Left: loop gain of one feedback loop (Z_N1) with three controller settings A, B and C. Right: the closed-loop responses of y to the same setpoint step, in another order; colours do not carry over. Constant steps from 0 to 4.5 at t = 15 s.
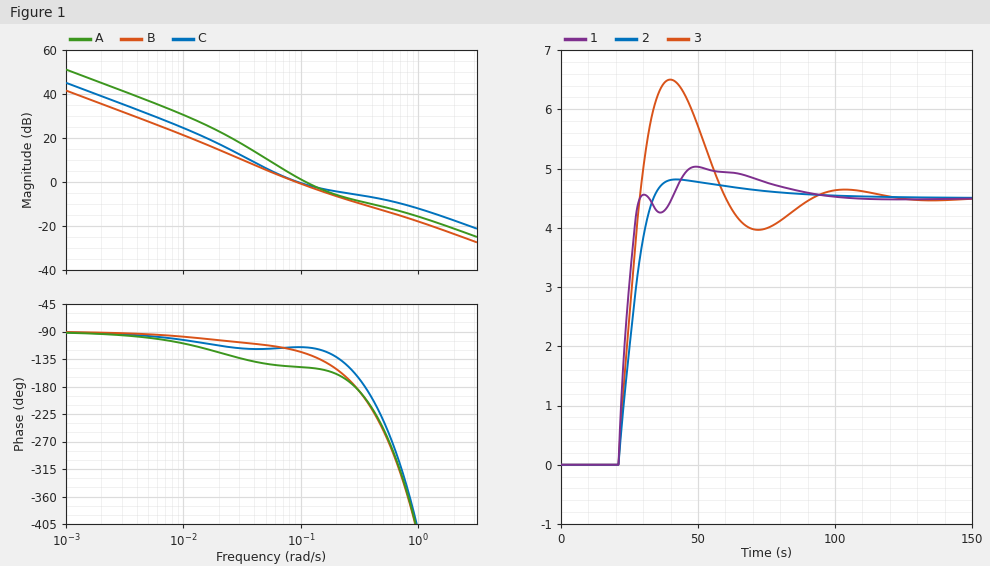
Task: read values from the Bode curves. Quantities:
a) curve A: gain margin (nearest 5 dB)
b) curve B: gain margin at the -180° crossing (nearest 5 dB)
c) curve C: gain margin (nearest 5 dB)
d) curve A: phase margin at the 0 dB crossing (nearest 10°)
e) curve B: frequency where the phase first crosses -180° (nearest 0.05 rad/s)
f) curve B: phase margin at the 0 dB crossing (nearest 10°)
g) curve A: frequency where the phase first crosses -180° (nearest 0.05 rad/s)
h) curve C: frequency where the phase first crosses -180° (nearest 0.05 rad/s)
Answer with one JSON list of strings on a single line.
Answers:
["10 dB", "10 dB", "5 dB", "30°", "0.30 rad/s", "60°", "0.30 rad/s", "0.35 rad/s"]
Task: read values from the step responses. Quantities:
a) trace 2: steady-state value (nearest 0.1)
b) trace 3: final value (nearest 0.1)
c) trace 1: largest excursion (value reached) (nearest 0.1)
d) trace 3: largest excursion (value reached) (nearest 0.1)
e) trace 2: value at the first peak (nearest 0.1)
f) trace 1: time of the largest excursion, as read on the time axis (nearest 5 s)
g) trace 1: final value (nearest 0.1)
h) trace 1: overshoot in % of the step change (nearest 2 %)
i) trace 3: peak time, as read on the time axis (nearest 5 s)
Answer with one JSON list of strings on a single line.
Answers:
["4.5", "4.5", "5.0", "6.5", "4.8", "50 s", "4.5", "12 %", "40 s"]
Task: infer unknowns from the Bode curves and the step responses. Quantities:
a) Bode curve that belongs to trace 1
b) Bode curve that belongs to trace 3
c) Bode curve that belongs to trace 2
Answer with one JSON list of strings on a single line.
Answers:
["C", "A", "B"]
